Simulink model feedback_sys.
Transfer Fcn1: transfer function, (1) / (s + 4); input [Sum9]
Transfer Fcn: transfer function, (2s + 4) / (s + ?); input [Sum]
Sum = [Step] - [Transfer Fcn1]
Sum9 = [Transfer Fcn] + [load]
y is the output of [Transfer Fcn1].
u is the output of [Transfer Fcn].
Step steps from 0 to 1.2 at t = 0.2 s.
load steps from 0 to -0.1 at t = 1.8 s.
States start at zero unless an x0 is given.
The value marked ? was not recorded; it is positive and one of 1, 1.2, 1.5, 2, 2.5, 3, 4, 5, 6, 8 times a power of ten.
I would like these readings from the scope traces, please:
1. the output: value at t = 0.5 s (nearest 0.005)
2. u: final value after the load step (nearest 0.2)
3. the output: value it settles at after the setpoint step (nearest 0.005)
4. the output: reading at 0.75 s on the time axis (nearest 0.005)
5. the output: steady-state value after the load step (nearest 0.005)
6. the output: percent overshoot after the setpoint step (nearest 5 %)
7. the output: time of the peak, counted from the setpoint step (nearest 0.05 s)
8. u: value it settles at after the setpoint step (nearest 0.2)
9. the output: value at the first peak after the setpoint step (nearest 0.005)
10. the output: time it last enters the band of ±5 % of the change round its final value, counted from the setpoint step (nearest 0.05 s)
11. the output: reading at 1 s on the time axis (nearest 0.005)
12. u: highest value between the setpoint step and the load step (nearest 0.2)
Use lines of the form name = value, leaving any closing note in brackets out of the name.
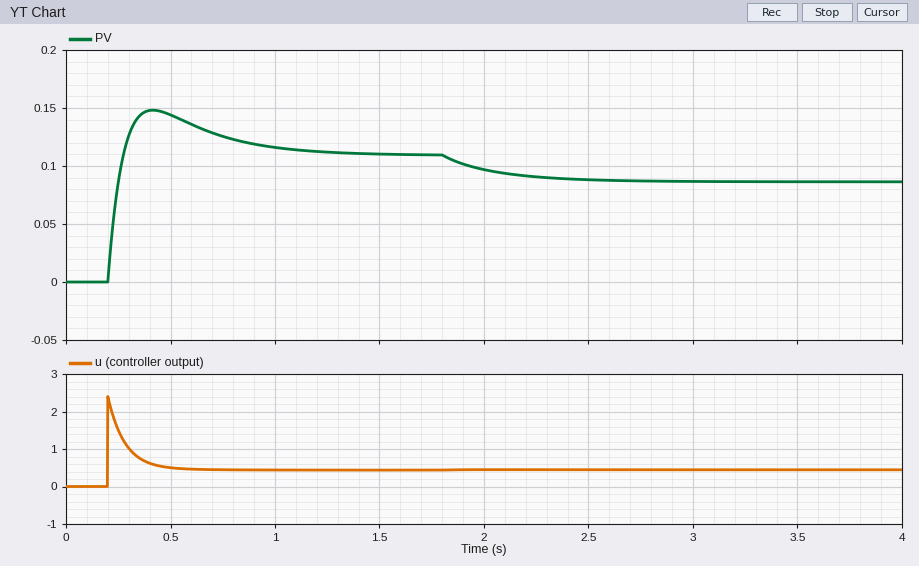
the output: value at t = 0.5 s = 0.145
u: final value after the load step = 0.4
the output: value it settles at after the setpoint step = 0.110
the output: reading at 0.75 s on the time axis = 0.125
the output: steady-state value after the load step = 0.085
the output: percent overshoot after the setpoint step = 35 %
the output: time of the peak, counted from the setpoint step = 0.20 s
u: value it settles at after the setpoint step = 0.4
the output: value at the first peak after the setpoint step = 0.150
the output: time it last enters the band of ±5 % of the change round its final value, counted from the setpoint step = 0.85 s
the output: reading at 1 s on the time axis = 0.115
u: highest value between the setpoint step and the load step = 2.4
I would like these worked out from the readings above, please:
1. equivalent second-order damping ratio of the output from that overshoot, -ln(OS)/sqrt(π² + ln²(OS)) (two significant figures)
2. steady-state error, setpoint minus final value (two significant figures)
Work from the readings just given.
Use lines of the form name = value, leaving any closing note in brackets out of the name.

equivalent second-order damping ratio of the output from that overshoot, -ln(OS)/sqrt(π² + ln²(OS)) = 0.32
steady-state error, setpoint minus final value = 1.1
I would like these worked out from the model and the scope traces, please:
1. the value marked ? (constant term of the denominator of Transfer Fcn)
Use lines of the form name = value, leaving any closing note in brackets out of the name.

the value marked ? = 10
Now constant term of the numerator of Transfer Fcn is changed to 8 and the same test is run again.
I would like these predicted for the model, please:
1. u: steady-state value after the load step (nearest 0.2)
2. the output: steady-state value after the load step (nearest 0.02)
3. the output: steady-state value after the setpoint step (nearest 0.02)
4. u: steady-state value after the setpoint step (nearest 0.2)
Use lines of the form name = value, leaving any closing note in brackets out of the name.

u: steady-state value after the load step = 0.8
the output: steady-state value after the load step = 0.18
the output: steady-state value after the setpoint step = 0.20
u: steady-state value after the setpoint step = 0.8
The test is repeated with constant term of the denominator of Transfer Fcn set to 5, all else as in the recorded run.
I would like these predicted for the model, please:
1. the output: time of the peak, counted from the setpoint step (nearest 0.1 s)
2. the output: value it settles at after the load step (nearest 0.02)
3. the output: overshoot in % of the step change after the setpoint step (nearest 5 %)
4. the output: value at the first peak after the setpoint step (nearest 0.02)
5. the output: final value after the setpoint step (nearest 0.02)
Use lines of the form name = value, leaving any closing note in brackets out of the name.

the output: time of the peak, counted from the setpoint step = 0.4 s
the output: value it settles at after the load step = 0.18
the output: overshoot in % of the step change after the setpoint step = 15 %
the output: value at the first peak after the setpoint step = 0.24
the output: final value after the setpoint step = 0.20
